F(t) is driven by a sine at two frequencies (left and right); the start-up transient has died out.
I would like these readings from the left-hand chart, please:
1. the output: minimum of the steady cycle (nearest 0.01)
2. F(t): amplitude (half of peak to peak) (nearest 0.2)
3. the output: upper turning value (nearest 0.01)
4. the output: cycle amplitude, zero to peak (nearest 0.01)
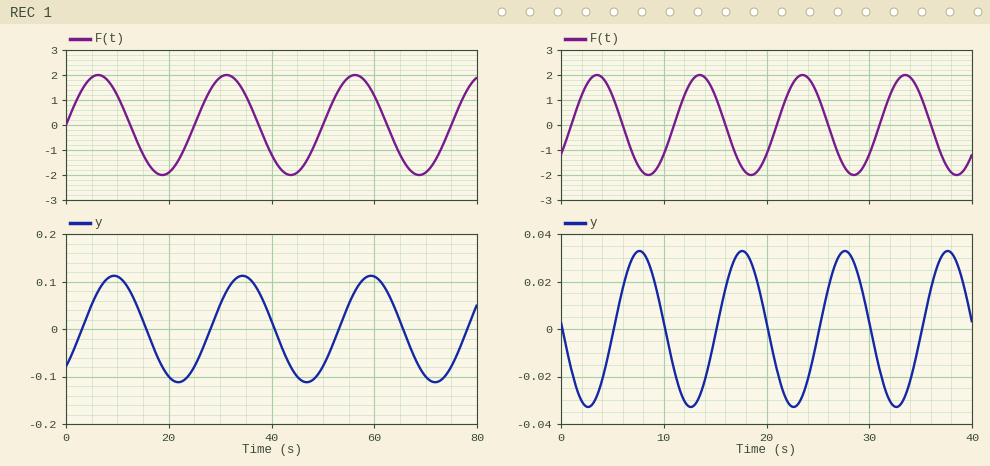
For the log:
-0.11
2.0
0.11
0.11
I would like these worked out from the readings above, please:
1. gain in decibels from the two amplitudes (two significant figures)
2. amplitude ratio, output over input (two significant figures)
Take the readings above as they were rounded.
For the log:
-25 dB
0.055
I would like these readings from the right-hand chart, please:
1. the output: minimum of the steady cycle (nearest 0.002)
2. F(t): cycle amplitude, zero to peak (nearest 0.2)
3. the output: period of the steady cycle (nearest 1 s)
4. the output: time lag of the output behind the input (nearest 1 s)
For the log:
-0.032
2.0
10 s
4 s
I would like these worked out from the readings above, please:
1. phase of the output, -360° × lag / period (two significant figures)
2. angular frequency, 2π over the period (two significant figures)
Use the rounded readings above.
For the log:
-140°
0.63 rad/s
